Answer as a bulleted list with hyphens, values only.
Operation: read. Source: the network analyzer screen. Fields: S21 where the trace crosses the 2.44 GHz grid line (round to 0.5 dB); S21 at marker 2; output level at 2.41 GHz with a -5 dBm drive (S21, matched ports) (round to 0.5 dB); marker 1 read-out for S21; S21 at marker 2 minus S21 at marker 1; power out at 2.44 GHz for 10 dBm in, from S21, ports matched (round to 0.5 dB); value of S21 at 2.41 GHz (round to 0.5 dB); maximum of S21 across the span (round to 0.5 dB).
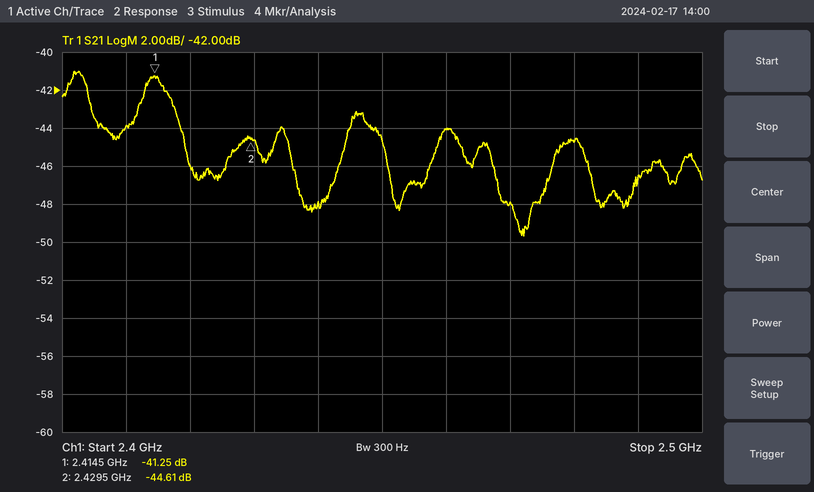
- -48.0 dB
- -44.61 dB
- -49.0 dBm
- -41.25 dB
- -3.36 dB
- -38.0 dBm
- -44.0 dB
- -41.0 dB
